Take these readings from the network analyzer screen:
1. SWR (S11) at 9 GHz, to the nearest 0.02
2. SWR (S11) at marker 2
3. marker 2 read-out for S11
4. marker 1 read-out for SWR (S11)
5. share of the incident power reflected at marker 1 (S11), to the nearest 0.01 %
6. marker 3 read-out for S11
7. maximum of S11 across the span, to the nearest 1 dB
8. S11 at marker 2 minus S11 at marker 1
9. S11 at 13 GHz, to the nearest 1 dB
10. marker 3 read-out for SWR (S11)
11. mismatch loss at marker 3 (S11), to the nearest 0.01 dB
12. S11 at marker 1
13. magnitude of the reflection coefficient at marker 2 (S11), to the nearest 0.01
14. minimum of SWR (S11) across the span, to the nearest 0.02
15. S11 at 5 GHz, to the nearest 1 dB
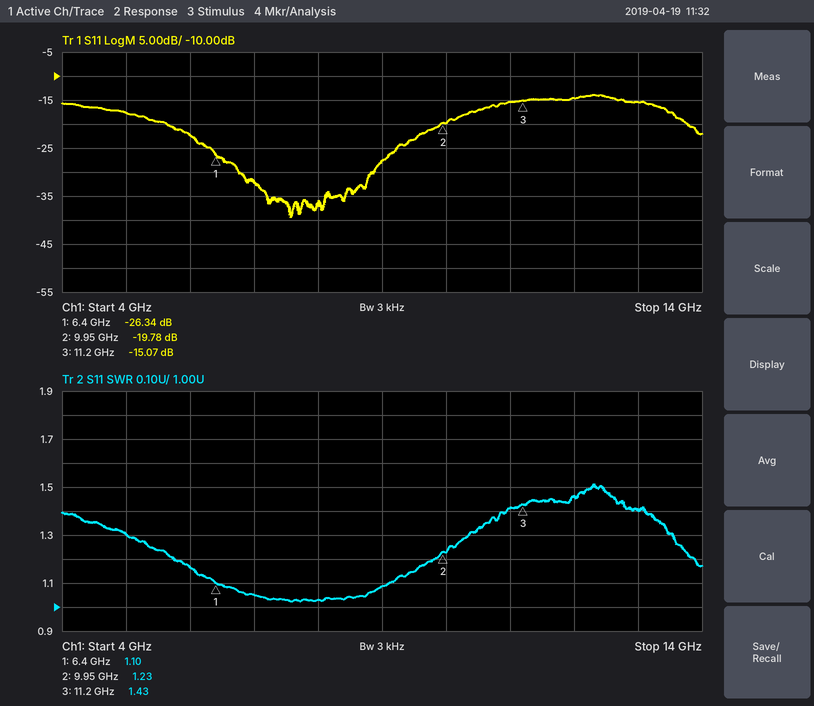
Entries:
1.08
1.23
-19.78 dB
1.10
0.23 %
-15.07 dB
-14 dB
6.56 dB
-15 dB
1.43
0.14 dB
-26.34 dB
0.10
1.02
-18 dB
